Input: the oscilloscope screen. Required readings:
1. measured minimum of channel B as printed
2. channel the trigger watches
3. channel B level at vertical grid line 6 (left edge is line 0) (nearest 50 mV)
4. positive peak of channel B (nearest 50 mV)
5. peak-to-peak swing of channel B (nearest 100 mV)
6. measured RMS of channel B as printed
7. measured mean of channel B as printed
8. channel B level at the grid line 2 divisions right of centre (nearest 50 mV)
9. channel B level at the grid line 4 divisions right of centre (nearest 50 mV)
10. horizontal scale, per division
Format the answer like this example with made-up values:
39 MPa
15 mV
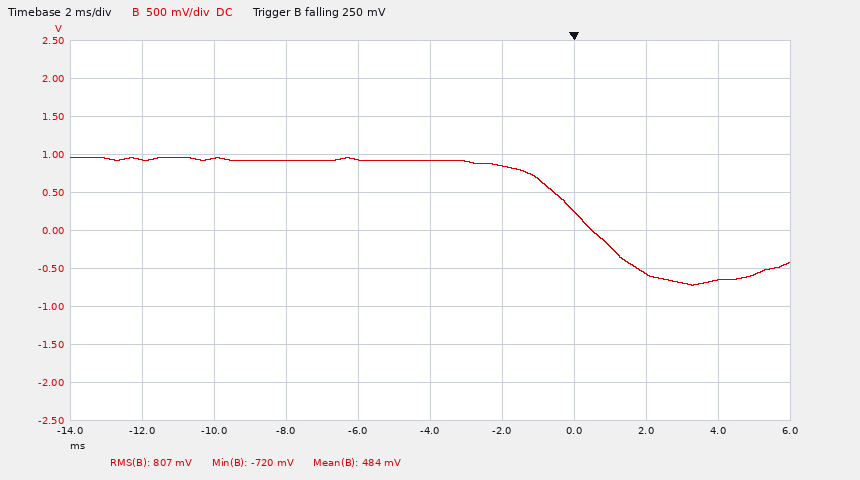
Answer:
-720 mV
channel B
850 mV
950 mV
1.70 V
807 mV
484 mV
250 mV
-650 mV
2 ms
